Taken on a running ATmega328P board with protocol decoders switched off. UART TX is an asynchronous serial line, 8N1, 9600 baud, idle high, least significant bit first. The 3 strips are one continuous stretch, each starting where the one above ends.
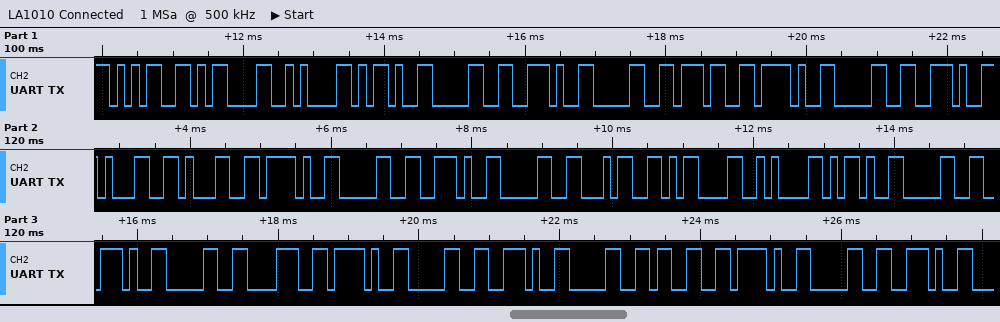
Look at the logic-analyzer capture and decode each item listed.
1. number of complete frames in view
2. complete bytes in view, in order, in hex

33
35 0D 0A 2D 30 2E 30 37 2F 30 2E 31 31 2F 30 2E 30 34 0D 0A 2D 30 2E 30 38 2F 30 2E 30 33 2F 30 2E
